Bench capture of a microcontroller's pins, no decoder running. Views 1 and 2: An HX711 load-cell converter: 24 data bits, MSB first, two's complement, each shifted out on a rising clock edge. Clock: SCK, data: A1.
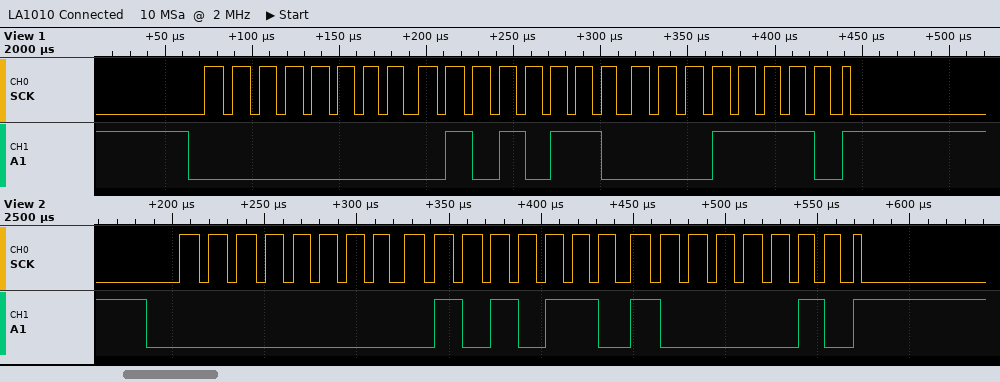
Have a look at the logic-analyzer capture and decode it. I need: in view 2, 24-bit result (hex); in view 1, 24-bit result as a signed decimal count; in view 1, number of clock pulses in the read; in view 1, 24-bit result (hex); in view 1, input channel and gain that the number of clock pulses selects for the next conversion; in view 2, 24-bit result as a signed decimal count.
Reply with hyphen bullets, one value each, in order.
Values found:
- 0x005682
- 22046
- 25
- 0x00561E
- channel A, gain 128
- 22146
